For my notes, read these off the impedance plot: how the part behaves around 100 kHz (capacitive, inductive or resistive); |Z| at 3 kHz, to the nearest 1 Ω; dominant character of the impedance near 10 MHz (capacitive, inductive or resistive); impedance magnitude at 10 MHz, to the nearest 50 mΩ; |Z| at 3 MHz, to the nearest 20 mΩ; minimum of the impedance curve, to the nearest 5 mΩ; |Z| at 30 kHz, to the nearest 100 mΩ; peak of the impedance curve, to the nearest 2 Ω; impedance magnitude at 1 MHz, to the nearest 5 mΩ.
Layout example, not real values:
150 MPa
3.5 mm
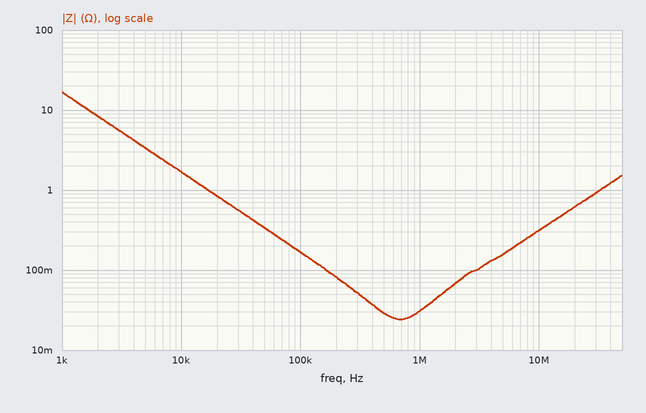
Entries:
capacitive
6 Ω
inductive
300 mΩ
100 mΩ
25 mΩ
600 mΩ
16 Ω
30 mΩ
